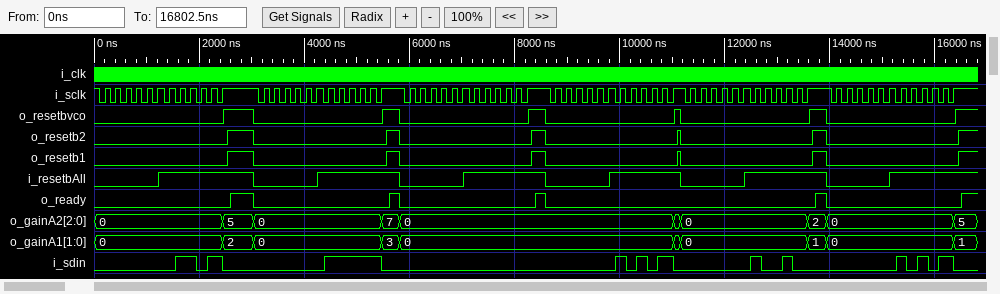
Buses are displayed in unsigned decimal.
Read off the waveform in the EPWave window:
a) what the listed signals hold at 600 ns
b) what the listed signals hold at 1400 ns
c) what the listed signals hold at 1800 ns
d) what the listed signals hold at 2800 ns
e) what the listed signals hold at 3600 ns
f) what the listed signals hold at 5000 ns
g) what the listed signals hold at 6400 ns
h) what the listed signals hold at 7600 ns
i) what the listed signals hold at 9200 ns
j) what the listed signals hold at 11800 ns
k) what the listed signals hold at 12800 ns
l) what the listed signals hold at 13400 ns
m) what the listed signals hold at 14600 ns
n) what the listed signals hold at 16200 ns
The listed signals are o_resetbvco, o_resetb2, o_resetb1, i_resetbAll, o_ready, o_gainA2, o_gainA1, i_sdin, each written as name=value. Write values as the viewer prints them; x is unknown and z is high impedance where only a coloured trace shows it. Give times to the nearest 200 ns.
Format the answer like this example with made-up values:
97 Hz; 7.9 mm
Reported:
o_resetbvco=0, o_resetb2=0, o_resetb1=0, i_resetbAll=0, o_ready=0, o_gainA2=0, o_gainA1=0, i_sdin=0; o_resetbvco=0, o_resetb2=0, o_resetb1=0, i_resetbAll=1, o_ready=0, o_gainA2=0, o_gainA1=0, i_sdin=0; o_resetbvco=0, o_resetb2=0, o_resetb1=0, i_resetbAll=1, o_ready=0, o_gainA2=0, o_gainA1=0, i_sdin=1; o_resetbvco=1, o_resetb2=1, o_resetb1=1, i_resetbAll=1, o_ready=1, o_gainA2=5, o_gainA1=2, i_sdin=0; o_resetbvco=0, o_resetb2=0, o_resetb1=0, i_resetbAll=0, o_ready=0, o_gainA2=0, o_gainA1=0, i_sdin=0; o_resetbvco=0, o_resetb2=0, o_resetb1=0, i_resetbAll=1, o_ready=0, o_gainA2=0, o_gainA1=0, i_sdin=1; o_resetbvco=0, o_resetb2=0, o_resetb1=0, i_resetbAll=0, o_ready=0, o_gainA2=0, o_gainA1=0, i_sdin=0; o_resetbvco=0, o_resetb2=0, o_resetb1=0, i_resetbAll=1, o_ready=0, o_gainA2=0, o_gainA1=0, i_sdin=0; o_resetbvco=0, o_resetb2=0, o_resetb1=0, i_resetbAll=0, o_ready=0, o_gainA2=0, o_gainA1=0, i_sdin=0; o_resetbvco=0, o_resetb2=0, o_resetb1=0, i_resetbAll=0, o_ready=0, o_gainA2=0, o_gainA1=0, i_sdin=0; o_resetbvco=0, o_resetb2=0, o_resetb1=0, i_resetbAll=1, o_ready=0, o_gainA2=0, o_gainA1=0, i_sdin=0; o_resetbvco=0, o_resetb2=0, o_resetb1=0, i_resetbAll=1, o_ready=0, o_gainA2=0, o_gainA1=0, i_sdin=0; o_resetbvco=0, o_resetb2=0, o_resetb1=0, i_resetbAll=0, o_ready=0, o_gainA2=0, o_gainA1=0, i_sdin=0; o_resetbvco=0, o_resetb2=0, o_resetb1=0, i_resetbAll=1, o_ready=0, o_gainA2=0, o_gainA1=0, i_sdin=1
